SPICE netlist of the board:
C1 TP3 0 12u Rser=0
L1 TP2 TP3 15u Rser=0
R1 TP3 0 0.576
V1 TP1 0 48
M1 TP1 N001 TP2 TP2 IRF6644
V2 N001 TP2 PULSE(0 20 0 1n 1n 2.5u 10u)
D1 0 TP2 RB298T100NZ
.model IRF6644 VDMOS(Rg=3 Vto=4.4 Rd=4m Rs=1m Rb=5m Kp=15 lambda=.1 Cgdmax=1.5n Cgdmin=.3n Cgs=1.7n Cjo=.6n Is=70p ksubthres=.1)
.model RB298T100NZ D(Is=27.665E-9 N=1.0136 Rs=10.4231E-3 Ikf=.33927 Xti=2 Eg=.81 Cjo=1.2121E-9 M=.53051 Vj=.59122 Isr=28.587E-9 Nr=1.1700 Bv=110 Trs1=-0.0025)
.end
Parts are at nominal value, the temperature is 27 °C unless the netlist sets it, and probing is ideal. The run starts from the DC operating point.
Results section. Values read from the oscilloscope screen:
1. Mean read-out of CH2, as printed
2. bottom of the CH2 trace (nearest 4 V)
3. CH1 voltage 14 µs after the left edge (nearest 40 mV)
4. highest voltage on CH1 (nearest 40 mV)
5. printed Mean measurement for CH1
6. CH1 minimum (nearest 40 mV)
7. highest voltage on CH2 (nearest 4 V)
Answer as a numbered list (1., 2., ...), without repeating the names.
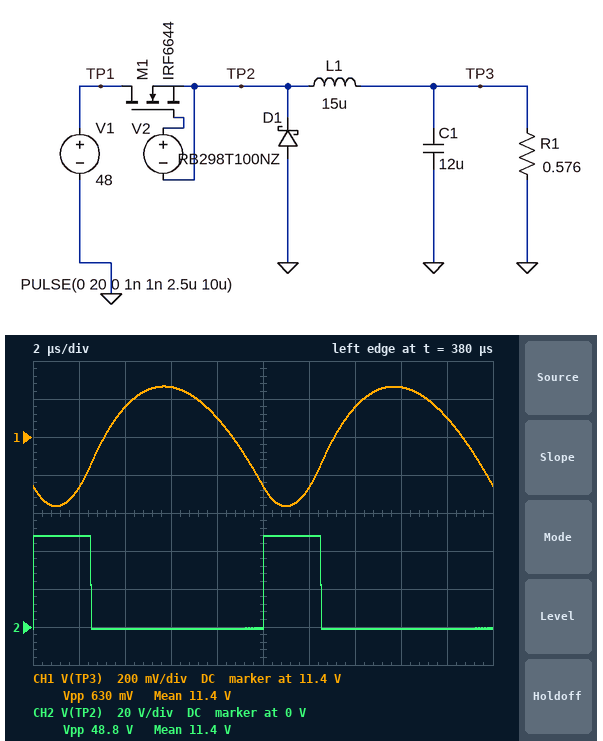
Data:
1. 11.4 V
2. 0 V
3. 11.56 V
4. 11.68 V
5. 11.4 V
6. 11.04 V
7. 48 V
